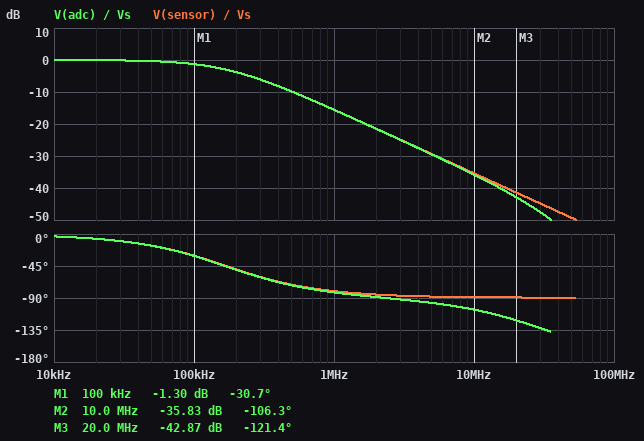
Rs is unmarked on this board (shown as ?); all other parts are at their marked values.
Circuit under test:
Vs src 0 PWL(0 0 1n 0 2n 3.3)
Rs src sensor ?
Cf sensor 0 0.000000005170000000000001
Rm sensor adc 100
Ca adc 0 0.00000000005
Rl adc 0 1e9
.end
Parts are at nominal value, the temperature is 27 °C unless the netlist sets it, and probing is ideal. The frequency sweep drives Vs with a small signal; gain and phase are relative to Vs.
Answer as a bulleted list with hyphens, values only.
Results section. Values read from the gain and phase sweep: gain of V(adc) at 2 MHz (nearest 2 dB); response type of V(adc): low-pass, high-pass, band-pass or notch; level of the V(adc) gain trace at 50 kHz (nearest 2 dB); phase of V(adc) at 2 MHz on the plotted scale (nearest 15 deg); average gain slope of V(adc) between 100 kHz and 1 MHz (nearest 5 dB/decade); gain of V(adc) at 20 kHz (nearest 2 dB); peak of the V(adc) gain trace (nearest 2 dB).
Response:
- -22 dB
- low-pass
- 0 dB
- -90 deg
- -15 dB/decade
- 0 dB
- 0 dB
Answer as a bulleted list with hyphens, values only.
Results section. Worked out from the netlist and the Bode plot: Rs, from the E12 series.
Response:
- 180 Ω
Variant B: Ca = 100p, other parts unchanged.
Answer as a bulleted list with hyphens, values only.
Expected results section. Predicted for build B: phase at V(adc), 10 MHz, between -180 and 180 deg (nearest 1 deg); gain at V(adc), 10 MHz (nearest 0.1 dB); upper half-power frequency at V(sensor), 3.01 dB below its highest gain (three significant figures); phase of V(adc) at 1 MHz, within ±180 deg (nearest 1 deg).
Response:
- -121 deg
- -36.9 dB
- 168 kHz
- -84 deg
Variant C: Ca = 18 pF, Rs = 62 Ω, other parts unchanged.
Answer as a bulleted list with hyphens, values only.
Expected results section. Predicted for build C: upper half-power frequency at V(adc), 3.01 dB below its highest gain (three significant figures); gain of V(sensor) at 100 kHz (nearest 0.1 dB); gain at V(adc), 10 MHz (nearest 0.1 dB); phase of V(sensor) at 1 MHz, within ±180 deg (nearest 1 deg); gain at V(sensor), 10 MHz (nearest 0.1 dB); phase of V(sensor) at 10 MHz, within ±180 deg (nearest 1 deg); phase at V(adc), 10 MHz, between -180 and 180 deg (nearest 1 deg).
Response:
- 495 kHz
- -0.2 dB
- -26.2 dB
- -64 deg
- -26.1 dB
- -87 deg
- -94 deg
